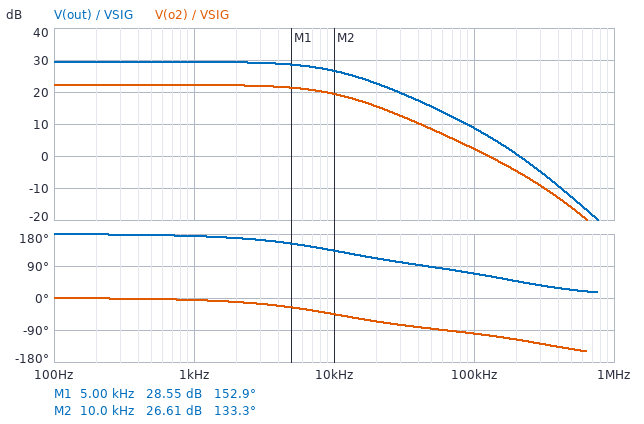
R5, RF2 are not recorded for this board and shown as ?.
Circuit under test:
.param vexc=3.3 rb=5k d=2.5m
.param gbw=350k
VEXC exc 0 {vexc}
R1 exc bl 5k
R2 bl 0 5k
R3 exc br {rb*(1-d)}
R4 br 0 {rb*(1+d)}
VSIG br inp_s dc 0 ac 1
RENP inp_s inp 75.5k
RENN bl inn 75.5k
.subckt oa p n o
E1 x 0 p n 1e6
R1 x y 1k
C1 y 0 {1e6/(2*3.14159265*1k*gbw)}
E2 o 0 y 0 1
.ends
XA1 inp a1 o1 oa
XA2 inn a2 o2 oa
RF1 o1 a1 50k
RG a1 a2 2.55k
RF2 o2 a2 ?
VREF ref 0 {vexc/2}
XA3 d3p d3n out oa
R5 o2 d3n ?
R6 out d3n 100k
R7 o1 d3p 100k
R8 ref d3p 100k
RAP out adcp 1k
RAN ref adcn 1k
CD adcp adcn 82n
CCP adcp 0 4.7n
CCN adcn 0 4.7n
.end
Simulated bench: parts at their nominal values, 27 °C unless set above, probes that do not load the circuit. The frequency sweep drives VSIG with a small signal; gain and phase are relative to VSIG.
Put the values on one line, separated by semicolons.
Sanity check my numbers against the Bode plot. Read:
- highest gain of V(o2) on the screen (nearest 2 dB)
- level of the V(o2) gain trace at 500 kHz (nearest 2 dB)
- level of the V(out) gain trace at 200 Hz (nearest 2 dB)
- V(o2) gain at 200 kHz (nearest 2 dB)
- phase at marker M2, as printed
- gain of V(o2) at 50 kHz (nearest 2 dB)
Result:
22 dB; -16 dB; 30 dB; -4 dB; 133.3 deg; 8 dB
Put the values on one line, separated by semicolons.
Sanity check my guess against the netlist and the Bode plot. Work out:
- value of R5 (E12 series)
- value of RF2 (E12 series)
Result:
120 kΩ; 33 kΩ
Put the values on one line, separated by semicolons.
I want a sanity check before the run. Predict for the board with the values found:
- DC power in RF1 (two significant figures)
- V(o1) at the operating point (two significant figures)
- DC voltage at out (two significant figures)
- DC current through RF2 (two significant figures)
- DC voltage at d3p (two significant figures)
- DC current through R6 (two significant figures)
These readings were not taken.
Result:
130 nW; 1.7 V; 1.8 V; 1.6 µA; 1.7 V; 800 nA
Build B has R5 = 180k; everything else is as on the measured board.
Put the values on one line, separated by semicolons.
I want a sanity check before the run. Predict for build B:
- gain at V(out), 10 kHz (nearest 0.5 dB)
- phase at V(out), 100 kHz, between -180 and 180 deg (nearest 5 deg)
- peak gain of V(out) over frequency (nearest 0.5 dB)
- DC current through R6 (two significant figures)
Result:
24.5 dB; 75 deg; 27.5 dB; 530 nA
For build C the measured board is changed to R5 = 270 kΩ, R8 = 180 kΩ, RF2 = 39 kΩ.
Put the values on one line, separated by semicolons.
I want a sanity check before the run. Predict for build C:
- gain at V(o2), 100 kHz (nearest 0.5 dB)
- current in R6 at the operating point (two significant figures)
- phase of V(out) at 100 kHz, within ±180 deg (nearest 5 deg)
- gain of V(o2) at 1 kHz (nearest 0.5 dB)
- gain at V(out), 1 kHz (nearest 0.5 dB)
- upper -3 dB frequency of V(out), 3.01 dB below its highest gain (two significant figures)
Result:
3.0 dB; 440 nA; 80 deg; 23.5 dB; 27.5 dB; 9.7 kHz
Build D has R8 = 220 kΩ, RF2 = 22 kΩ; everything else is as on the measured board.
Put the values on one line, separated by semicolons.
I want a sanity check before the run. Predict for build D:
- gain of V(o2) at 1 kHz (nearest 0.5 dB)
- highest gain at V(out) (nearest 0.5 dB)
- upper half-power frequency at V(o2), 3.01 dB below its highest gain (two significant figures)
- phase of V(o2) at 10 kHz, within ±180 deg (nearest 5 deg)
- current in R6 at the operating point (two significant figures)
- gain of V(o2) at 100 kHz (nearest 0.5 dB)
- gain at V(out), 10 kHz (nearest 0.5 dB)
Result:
18.5 dB; 30.5 dB; 12 kHz; -40 deg; 780 nA; 0 dB; 28.0 dB
